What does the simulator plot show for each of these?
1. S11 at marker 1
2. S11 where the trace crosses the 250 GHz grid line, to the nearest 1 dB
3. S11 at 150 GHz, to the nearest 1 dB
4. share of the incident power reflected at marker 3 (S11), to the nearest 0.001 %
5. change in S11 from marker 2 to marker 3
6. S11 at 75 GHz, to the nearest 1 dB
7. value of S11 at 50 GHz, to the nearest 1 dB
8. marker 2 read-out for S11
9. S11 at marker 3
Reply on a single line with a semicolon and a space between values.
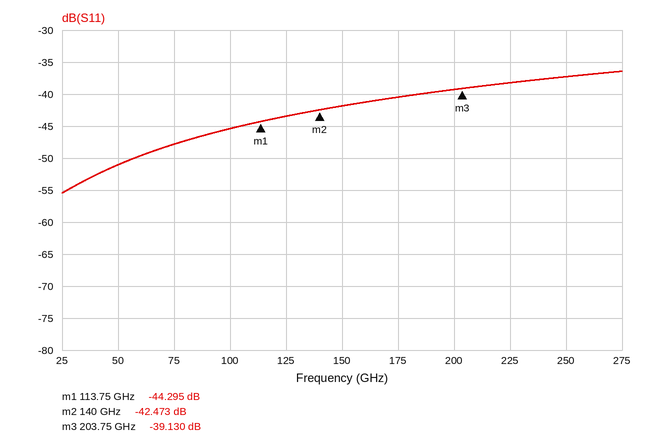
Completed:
-44.295 dB; -37 dB; -42 dB; 0.012 %; 3.343 dB; -48 dB; -51 dB; -42.473 dB; -39.130 dB
